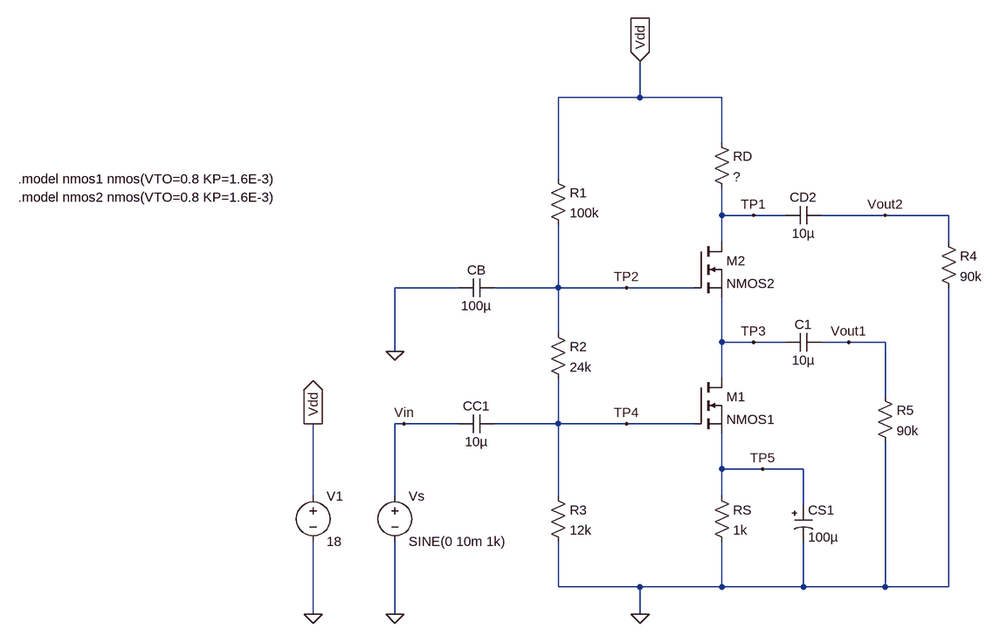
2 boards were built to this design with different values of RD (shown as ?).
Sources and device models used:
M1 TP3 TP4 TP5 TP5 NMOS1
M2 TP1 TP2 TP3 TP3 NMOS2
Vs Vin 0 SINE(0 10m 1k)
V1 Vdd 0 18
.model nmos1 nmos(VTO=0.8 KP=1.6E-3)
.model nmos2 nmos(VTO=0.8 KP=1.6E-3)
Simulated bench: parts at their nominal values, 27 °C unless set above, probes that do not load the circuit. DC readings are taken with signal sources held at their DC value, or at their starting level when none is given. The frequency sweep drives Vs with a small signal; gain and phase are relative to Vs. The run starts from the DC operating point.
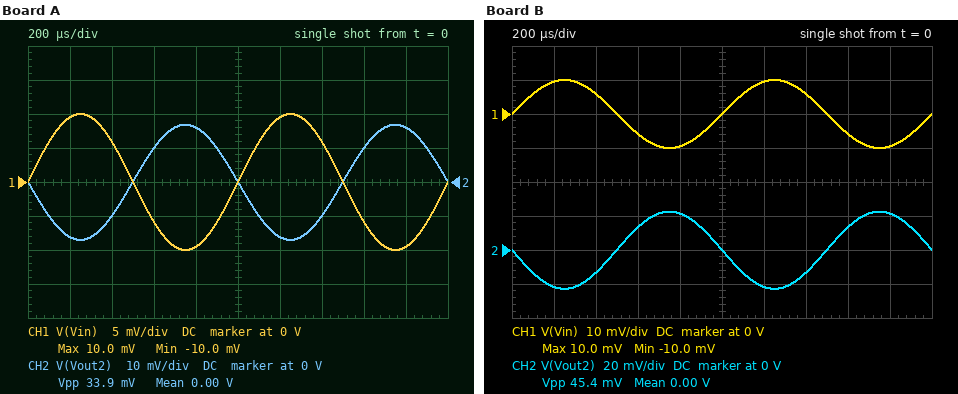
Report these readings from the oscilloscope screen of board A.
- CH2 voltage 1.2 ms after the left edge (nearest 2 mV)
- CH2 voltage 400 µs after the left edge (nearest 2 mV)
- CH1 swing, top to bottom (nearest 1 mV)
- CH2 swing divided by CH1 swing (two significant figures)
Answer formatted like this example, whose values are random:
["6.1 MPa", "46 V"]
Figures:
["-16 mV", "-10 mV", "20 mV", "1.7"]
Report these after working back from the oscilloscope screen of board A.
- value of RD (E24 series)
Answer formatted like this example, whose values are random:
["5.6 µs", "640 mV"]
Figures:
["2 kΩ"]
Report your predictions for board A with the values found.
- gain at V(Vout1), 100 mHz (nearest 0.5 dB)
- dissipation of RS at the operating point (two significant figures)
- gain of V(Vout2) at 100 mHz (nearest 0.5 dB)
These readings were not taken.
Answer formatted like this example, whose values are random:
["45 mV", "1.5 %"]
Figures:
["-38.0 dB", "58 µW", "-32.0 dB"]
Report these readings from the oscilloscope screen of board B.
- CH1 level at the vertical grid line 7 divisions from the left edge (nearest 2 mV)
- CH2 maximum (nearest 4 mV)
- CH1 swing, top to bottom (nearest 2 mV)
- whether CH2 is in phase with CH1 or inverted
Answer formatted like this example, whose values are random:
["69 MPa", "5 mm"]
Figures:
["6 mV", "24 mV", "20 mV", "inverted"]
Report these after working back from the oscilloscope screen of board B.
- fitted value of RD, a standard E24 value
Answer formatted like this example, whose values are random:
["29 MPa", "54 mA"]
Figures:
["2.7 kΩ"]
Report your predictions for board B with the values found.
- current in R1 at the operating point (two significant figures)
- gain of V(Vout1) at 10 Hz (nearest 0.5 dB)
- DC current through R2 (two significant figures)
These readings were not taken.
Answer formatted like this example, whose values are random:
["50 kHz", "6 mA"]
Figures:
["130 µA", "-0.5 dB", "130 µA"]
